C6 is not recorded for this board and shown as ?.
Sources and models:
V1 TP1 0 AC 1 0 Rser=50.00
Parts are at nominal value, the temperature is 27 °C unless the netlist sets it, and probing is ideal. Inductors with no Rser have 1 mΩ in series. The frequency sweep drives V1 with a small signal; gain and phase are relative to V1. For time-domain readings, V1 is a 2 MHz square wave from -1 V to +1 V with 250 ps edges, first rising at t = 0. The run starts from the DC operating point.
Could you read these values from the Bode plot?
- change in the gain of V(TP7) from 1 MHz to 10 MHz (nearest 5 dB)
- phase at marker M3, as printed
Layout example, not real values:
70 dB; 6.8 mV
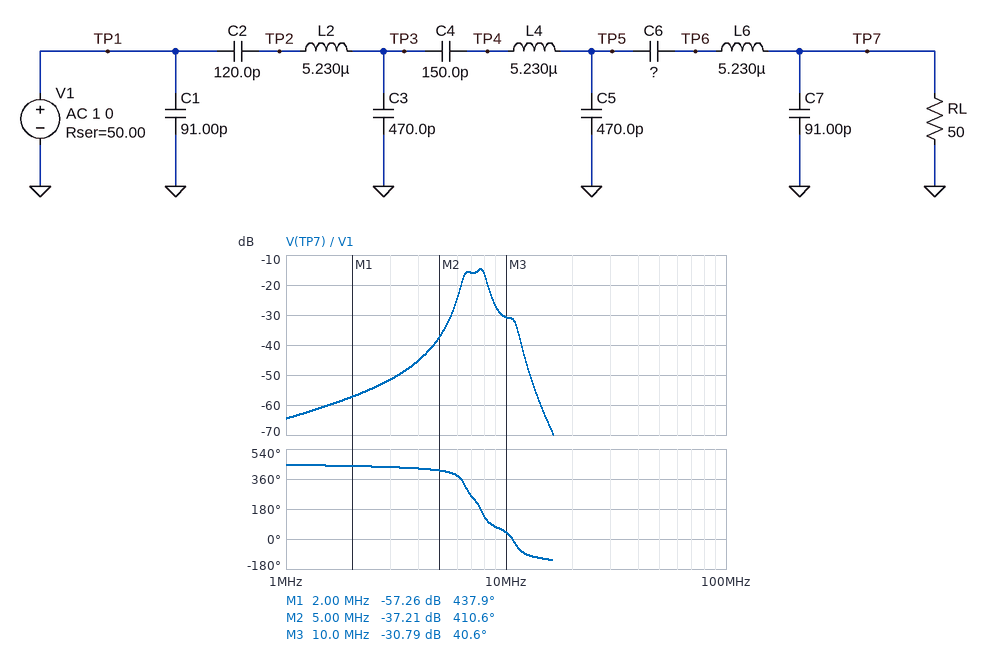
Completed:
35 dB; 40.6 deg
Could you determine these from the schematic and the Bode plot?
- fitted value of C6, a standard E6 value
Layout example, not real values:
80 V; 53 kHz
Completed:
47 pF
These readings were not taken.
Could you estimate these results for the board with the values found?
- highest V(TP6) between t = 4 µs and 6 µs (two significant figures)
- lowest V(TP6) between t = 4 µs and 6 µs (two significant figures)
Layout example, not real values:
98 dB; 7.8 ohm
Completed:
150 mV; -150 mV
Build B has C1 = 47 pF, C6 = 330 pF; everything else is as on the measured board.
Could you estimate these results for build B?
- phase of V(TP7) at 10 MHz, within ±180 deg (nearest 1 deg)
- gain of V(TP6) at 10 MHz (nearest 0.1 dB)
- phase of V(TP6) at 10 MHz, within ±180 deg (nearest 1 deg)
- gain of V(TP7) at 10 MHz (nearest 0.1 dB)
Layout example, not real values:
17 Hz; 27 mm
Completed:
-84 deg; -23.7 dB; 13 deg; -40.1 dB
